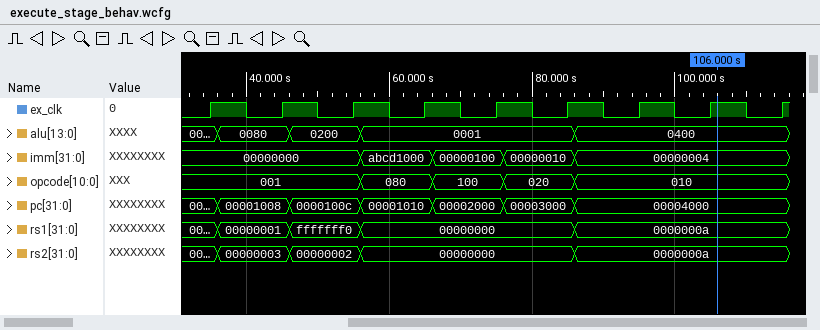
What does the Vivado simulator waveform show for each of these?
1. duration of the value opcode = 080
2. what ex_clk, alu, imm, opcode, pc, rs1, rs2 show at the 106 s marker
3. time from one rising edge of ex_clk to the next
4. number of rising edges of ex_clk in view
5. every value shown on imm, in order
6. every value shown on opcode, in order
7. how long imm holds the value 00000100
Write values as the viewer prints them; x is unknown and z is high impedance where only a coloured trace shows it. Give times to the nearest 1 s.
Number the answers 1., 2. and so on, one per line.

1. 10 s
2. ex_clk=1, alu=0400, imm=00000004, opcode=010, pc=00004000, rs1=0000000a, rs2=0000000a
3. 10 s
4. 9
5. 00000000, abcd1000, 00000100, 00000010, 00000004
6. 001, 080, 100, 020, 010
7. 10 s
